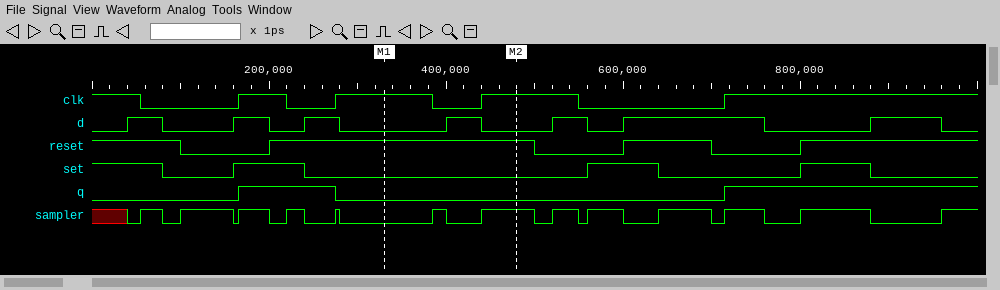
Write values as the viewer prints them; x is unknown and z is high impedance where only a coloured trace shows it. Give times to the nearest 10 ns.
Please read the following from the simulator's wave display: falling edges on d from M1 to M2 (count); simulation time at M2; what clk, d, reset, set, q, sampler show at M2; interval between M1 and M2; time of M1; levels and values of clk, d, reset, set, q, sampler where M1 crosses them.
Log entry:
1
480 ns
clk=1, d=0, reset=1, set=0, q=0, sampler=1
150 ns
330 ns
clk=1, d=0, reset=1, set=0, q=0, sampler=0
